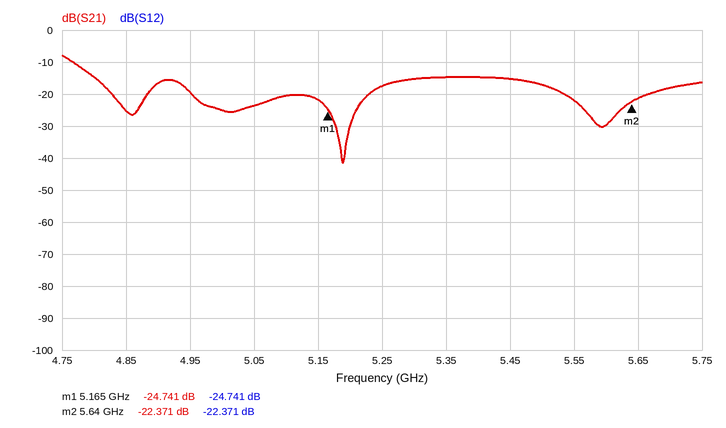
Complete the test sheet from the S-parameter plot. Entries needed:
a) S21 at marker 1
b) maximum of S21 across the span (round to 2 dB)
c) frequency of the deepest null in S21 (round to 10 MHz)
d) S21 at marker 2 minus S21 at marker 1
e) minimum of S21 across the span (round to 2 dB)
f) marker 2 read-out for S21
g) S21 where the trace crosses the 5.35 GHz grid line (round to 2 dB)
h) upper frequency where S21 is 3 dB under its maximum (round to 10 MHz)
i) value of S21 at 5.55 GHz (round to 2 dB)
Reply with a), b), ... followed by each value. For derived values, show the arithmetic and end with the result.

a) -24.741 dB
b) -8 dB
c) 5.19 GHz
d) -22.371 − (-24.741) = 2.370 dB
e) -42 dB
f) -22.371 dB
g) -14 dB
h) 4.77 GHz
i) -22 dB
